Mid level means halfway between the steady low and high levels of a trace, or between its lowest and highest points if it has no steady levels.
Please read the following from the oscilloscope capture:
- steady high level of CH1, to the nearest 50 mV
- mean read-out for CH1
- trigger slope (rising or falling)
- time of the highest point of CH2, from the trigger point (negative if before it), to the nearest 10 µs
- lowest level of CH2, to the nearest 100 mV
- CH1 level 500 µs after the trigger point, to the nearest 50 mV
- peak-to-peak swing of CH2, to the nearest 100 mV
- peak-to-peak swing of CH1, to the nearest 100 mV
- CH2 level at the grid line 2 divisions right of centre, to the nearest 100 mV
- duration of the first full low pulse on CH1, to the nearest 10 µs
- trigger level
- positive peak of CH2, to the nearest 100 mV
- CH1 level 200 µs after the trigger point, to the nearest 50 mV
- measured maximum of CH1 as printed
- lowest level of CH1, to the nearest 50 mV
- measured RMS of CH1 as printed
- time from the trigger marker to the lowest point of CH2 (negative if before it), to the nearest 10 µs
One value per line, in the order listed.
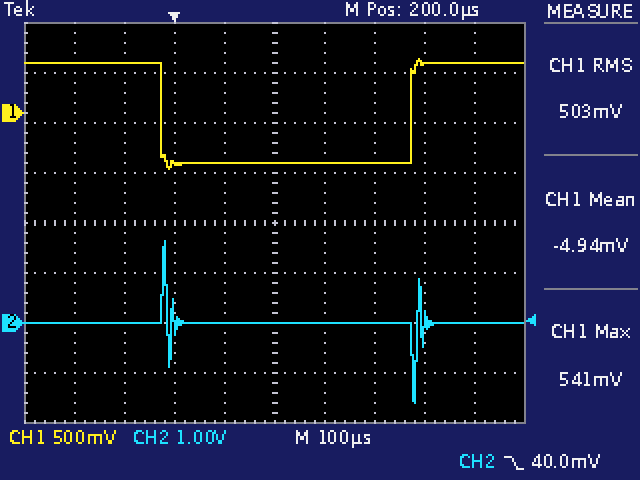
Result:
500 mV
-4.94 mV
falling
-20 µs
-1.6 V
500 mV
3.2 V
1.10 V
0.0 V
500 µs
40.0 mV
1.6 V
-500 mV
541 mV
-550 mV
503 mV
+480 µs
